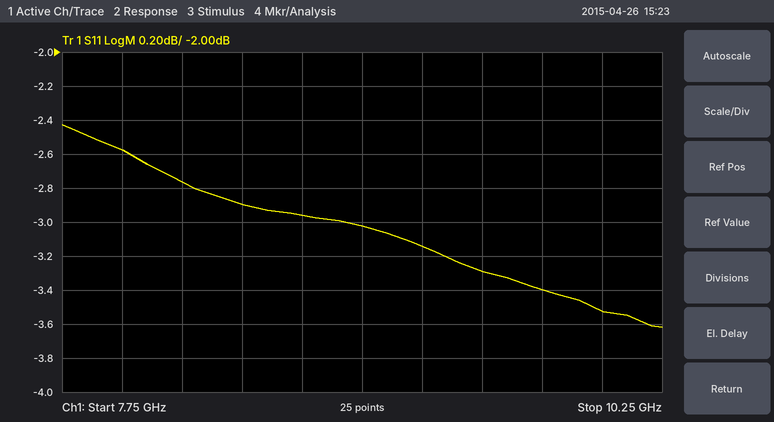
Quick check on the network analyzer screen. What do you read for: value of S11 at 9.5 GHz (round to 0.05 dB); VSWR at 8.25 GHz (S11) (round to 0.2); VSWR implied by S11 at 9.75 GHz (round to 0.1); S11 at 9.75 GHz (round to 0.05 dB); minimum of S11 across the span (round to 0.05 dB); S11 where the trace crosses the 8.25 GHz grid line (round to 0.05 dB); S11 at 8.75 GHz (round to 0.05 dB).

-3.30 dB
6.4
5.2
-3.40 dB
-3.60 dB
-2.75 dB
-2.95 dB
